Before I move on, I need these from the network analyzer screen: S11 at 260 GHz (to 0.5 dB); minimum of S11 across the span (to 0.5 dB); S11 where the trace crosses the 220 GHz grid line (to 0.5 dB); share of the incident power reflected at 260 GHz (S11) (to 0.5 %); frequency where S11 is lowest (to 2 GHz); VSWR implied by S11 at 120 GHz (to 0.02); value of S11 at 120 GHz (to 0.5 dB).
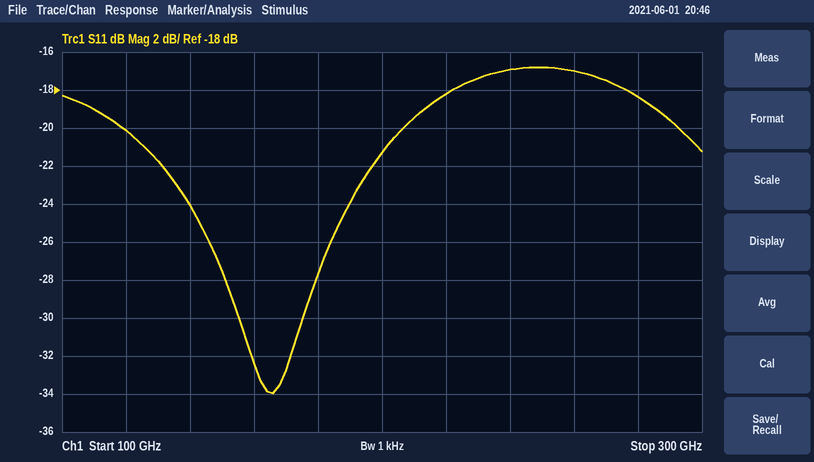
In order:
-17.0 dB
-34.0 dB
-18.0 dB
2.0 %
166 GHz
1.22
-20.0 dB
